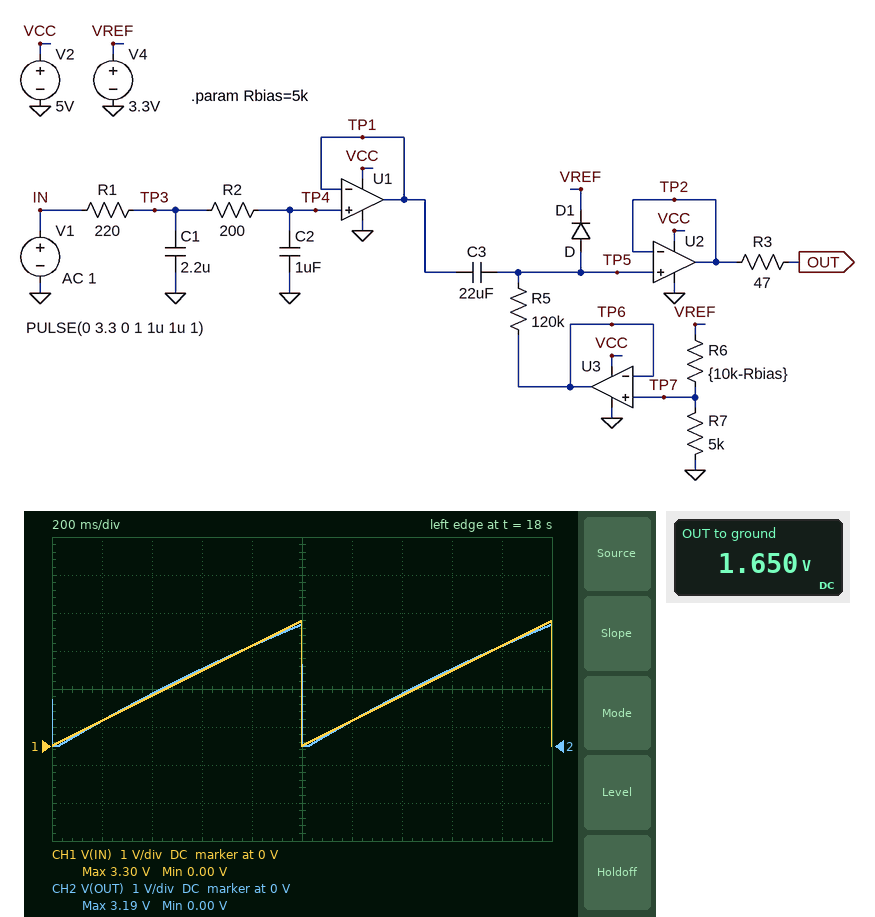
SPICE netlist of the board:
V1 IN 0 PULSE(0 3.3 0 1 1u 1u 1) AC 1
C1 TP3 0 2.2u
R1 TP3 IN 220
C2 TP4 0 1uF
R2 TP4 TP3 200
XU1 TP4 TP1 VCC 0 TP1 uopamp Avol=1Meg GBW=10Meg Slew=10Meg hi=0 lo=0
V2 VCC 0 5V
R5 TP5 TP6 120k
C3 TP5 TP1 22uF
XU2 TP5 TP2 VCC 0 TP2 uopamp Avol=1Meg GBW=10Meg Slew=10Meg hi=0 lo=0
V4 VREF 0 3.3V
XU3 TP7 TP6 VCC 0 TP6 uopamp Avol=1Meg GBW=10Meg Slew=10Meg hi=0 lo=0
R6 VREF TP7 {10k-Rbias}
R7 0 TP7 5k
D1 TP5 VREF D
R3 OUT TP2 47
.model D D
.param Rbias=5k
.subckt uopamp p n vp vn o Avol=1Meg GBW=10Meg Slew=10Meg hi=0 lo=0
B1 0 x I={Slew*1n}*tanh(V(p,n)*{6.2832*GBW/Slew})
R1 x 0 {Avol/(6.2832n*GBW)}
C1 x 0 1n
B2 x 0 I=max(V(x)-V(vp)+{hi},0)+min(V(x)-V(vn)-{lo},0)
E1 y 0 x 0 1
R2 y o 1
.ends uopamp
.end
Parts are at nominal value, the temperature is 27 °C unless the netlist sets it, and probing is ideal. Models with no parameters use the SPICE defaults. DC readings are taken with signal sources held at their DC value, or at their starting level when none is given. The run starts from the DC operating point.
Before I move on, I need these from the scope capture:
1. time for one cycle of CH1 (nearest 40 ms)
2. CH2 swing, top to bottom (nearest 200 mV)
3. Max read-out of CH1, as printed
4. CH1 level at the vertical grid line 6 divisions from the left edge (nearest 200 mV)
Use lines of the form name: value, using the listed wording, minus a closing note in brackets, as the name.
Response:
time for one cycle of CH1: 1.00 s
CH2 swing, top to bottom: 3.2 V
Max read-out of CH1, as printed: 3.30 V
CH1 level at the vertical grid line 6 divisions from the left edge: 600 mV
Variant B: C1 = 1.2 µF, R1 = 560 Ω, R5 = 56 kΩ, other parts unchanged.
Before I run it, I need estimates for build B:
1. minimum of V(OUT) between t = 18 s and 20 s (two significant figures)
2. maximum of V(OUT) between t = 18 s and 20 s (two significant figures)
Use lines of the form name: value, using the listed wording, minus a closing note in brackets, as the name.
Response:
minimum of V(OUT) between t = 18 s and 20 s: -8.0 mV
maximum of V(OUT) between t = 18 s and 20 s: 3.1 V
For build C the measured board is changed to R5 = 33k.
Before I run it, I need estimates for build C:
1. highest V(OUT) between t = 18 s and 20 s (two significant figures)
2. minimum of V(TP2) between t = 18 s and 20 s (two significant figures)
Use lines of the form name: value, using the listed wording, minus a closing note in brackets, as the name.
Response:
highest V(OUT) between t = 18 s and 20 s: 2.9 V
minimum of V(TP2) between t = 18 s and 20 s: -9.7 mV
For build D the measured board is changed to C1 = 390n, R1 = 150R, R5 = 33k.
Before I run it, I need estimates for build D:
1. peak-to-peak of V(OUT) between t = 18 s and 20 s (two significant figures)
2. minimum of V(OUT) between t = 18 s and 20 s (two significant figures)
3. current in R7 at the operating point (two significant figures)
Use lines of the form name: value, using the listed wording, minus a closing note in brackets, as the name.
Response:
peak-to-peak of V(OUT) between t = 18 s and 20 s: 2.9 V
minimum of V(OUT) between t = 18 s and 20 s: -9.7 mV
current in R7 at the operating point: 330 µA
